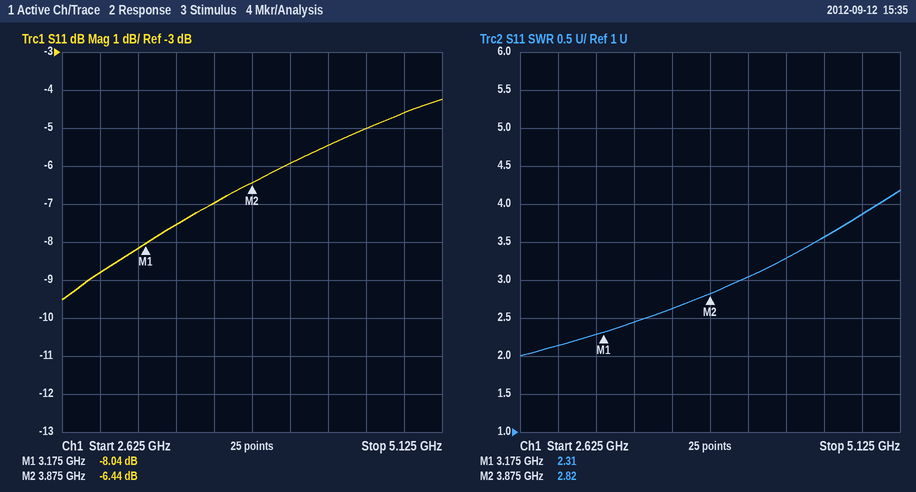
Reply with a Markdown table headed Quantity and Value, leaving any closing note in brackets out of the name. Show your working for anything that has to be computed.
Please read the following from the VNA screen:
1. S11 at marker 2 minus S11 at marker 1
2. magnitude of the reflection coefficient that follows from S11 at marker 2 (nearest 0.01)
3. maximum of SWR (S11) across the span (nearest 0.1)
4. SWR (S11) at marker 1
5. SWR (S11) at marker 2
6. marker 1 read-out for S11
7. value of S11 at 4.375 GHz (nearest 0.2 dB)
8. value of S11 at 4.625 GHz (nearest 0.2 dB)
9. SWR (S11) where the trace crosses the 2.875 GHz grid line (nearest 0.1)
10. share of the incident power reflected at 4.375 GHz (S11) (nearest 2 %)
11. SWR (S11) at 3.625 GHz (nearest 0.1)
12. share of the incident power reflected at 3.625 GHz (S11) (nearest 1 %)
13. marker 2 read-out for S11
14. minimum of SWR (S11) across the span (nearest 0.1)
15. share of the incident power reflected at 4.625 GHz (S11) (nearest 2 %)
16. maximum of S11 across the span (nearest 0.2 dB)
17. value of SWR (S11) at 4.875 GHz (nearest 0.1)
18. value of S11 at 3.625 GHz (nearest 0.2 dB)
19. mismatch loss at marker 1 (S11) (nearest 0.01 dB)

| Quantity | Value |
|---|---|
| S11 at marker 2 minus S11 at marker 1 | -6.44 − (-8.04) = 1.60 dB |
| magnitude of the reflection coefficient that follows from S11 at marker 2 | 10^(-6.44/20) ≈ 0.48 |
| maximum of SWR (S11) across the span | 4.2 |
| SWR (S11) at marker 1 | 2.31 |
| SWR (S11) at marker 2 | 2.82 |
| marker 1 read-out for S11 | -8.04 dB |
| value of S11 at 4.375 GHz | -5.4 dB |
| value of S11 at 4.625 GHz | -5.0 dB |
| SWR (S11) where the trace crosses the 2.875 GHz grid line | 2.1 |
| share of the incident power reflected at 4.375 GHz (S11) | 10^(-5.4/10) ≈ 28.8 %, so 28 % to the nearest 2 % |
| SWR (S11) at 3.625 GHz | 2.6 |
| share of the incident power reflected at 3.625 GHz (S11) | 10^(-7/10) ≈ 20 % |
| marker 2 read-out for S11 | -6.44 dB |
| minimum of SWR (S11) across the span | 2.0 |
| share of the incident power reflected at 4.625 GHz (S11) | 10^(-5/10) ≈ 32 % |
| maximum of S11 across the span | -4.2 dB |
| value of SWR (S11) at 4.875 GHz | 3.9 |
| value of S11 at 3.625 GHz | -7.0 dB |
| mismatch loss at marker 1 (S11) | −10 log10(1 − 10^(-8.04/10)) ≈ 0.74 dB |
